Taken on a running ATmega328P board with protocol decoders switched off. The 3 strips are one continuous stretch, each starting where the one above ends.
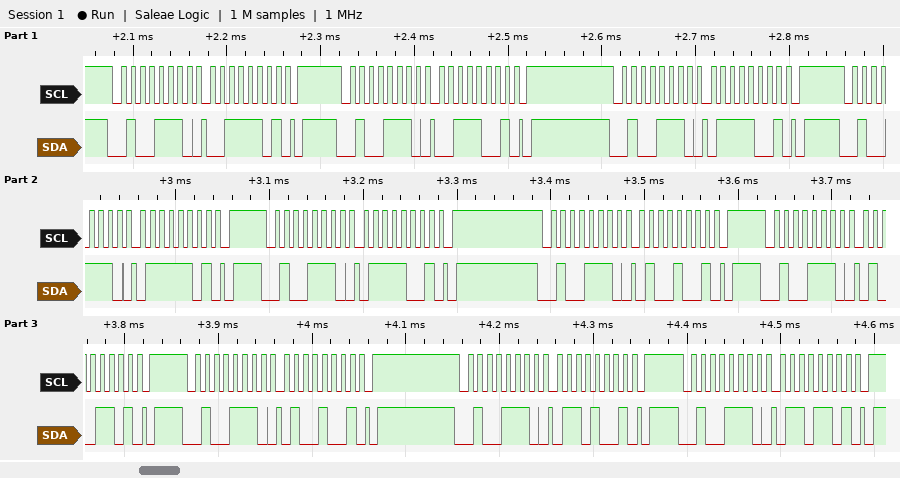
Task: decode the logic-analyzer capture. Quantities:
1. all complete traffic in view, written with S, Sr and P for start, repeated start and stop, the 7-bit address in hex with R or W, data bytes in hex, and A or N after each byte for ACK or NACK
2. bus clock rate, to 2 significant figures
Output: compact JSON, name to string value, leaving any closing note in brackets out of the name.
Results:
{"all complete traffic in view, written with S, Sr and P for start, repeated start and stop, the 7-bit address in hex with R or W, data bytes in hex, and A or N after each byte for ACK or NACK": "S 27W A 3D A P S 27W A 39 A P S 27W A 79 A P S 27W A 7D A P S 27W A 79 A P S 27W A 49 A P S 27W A 4D A P S 27W A 49 A P S 27W A 69 A P S 27W A 6D A P", "bus clock rate, to 2 significant figures": "100 kHz"}
